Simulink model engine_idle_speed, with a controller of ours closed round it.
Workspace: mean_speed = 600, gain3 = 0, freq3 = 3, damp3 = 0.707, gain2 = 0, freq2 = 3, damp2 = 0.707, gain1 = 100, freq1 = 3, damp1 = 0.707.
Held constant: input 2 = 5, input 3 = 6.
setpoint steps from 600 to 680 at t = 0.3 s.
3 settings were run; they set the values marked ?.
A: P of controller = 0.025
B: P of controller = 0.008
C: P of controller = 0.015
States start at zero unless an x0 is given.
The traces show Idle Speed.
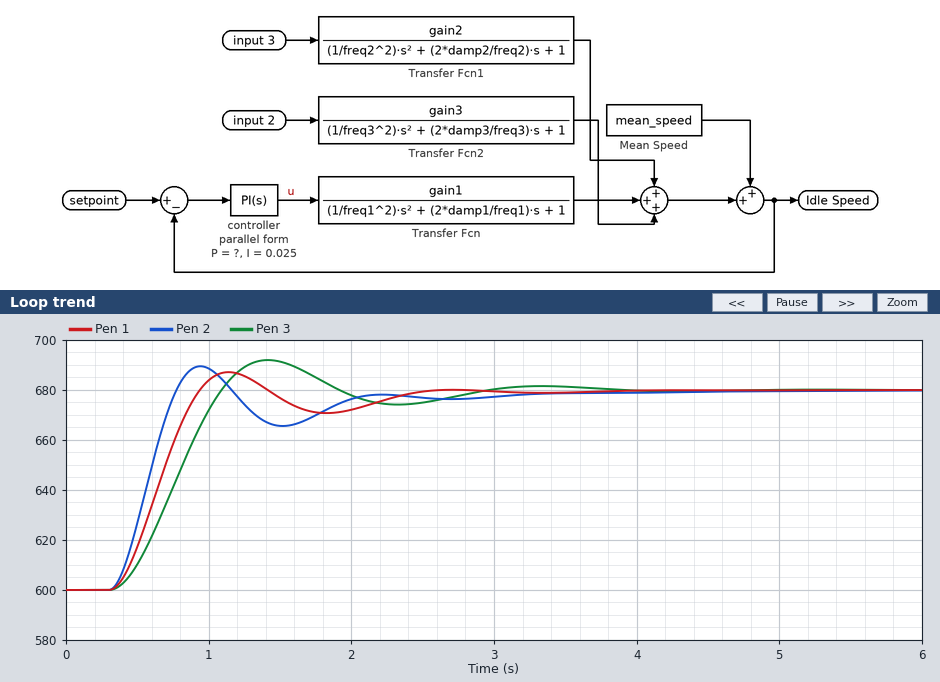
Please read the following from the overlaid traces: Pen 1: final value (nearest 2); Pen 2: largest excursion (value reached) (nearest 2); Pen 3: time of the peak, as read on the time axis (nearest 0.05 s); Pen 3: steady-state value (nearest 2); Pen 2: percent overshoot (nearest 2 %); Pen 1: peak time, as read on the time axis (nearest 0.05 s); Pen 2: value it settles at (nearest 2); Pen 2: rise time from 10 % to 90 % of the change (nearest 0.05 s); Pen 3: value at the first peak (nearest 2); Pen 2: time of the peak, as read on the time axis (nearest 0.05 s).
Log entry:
680
690
1.40 s
680
12 %
1.15 s
680
0.30 s
692
0.95 s
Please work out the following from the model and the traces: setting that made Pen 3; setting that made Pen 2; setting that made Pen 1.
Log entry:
B
A
C
